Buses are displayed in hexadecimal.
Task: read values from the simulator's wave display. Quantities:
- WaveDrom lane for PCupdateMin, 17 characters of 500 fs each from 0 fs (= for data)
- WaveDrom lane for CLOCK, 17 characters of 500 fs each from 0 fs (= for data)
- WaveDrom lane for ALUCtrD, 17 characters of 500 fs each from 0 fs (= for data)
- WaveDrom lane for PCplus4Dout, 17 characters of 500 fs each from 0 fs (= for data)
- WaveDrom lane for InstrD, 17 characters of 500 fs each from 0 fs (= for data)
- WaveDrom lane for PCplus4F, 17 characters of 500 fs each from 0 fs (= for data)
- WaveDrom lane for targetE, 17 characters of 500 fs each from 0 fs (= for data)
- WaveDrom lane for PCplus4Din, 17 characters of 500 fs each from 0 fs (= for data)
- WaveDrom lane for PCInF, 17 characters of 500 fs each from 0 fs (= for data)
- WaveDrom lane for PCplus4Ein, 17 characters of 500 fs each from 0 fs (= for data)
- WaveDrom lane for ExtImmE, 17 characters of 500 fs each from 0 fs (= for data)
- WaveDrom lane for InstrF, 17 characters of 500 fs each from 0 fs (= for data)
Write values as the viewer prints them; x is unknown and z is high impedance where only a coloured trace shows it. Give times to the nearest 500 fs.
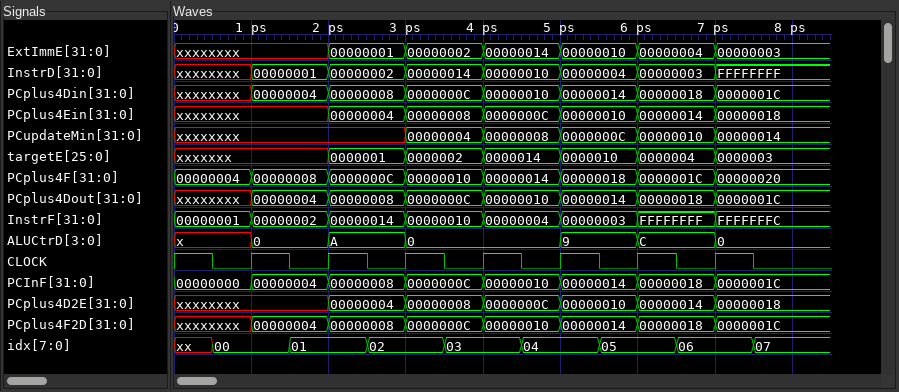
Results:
{name: 'PCupdateMin', wave: 'x.....=.=.=.=.=..', data: '00000004 00000008 0000000C 00000010 00000014'}
{name: 'CLOCK', wave: '1010101010101010.'}
{name: 'ALUCtrD', wave: 'x.=.=.=...=.=.=..', data: '0 A 0 9 C 0'}
{name: 'PCplus4Dout', wave: 'x.=.=.=.=.=.=.=..', data: '00000004 00000008 0000000C 00000010 00000014 00000018 0000001C'}
{name: 'InstrD', wave: 'x.=.=.=.=.=.=.=..', data: '00000001 00000002 00000014 00000010 00000004 00000003 FFFFFFFF'}
{name: 'PCplus4F', wave: '=.=.=.=.=.=.=.=..', data: '00000004 00000008 0000000C 00000010 00000014 00000018 0000001C 00000020'}
{name: 'targetE', wave: 'x...=.=.=.=.=.=..', data: '0000001 0000002 0000014 0000010 0000004 0000003'}
{name: 'PCplus4Din', wave: 'x.=.=.=.=.=.=.=..', data: '00000004 00000008 0000000C 00000010 00000014 00000018 0000001C'}
{name: 'PCInF', wave: '=.=.=.=.=.=.=.=..', data: '00000000 00000004 00000008 0000000C 00000010 00000014 00000018 0000001C'}
{name: 'PCplus4Ein', wave: 'x...=.=.=.=.=.=..', data: '00000004 00000008 0000000C 00000010 00000014 00000018'}
{name: 'ExtImmE', wave: 'x...=.=.=.=.=.=..', data: '00000001 00000002 00000014 00000010 00000004 00000003'}
{name: 'InstrF', wave: '=.=.=.=.=.=.=.=..', data: '00000001 00000002 00000014 00000010 00000004 00000003 FFFFFFFF FFFFFFFC'}
